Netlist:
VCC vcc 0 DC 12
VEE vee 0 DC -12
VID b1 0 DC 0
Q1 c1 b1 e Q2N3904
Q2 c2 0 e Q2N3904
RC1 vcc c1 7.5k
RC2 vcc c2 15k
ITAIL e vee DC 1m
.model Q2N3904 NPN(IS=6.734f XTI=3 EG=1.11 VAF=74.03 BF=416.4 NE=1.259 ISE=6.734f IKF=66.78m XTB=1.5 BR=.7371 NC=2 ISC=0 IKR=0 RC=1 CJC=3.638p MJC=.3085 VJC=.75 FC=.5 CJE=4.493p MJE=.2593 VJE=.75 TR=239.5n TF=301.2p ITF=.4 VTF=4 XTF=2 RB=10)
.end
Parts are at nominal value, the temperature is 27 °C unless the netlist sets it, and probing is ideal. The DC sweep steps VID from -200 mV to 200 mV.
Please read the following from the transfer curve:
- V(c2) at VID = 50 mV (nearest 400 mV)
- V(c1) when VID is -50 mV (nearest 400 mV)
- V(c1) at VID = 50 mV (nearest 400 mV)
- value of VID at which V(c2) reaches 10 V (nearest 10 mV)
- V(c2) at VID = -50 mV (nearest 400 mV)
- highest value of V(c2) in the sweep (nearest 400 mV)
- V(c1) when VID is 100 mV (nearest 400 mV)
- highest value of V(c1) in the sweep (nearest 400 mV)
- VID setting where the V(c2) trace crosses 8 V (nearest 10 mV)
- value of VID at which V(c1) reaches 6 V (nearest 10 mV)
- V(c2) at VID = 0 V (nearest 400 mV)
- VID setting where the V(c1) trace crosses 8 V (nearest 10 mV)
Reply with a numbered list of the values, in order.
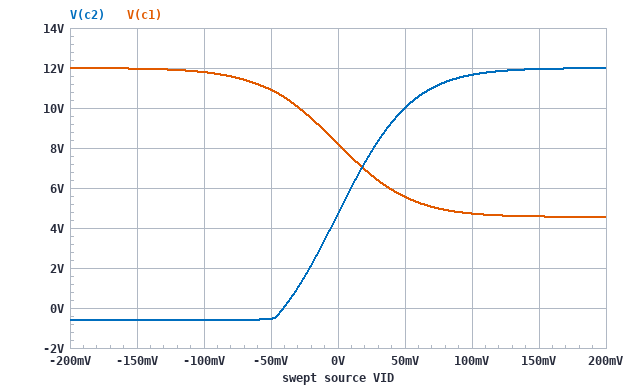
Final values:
1. 10.0 V
2. 10.8 V
3. 5.6 V
4. 50 mV
5. -400 mV
6. 12.0 V
7. 4.8 V
8. 12.0 V
9. 30 mV
10. 40 mV
11. 4.8 V
12. 0 V
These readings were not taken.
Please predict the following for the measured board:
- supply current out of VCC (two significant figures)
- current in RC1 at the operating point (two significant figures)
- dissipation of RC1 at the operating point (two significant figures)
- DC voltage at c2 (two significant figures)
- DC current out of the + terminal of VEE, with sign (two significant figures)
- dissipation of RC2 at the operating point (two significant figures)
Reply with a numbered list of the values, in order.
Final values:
1. 990 µA
2. 510 µA
3. 1.9 mW
4. 4.7 V
5. -1.0 mA
6. 3.5 mW
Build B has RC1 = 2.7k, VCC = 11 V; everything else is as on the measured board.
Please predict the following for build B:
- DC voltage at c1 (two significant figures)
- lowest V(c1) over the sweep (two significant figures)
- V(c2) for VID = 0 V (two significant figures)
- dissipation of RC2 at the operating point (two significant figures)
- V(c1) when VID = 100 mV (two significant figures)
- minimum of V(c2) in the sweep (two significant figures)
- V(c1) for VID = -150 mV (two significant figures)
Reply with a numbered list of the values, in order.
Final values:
1. 9.6 V
2. 8.3 V
3. 3.8 V
4. 3.4 mW
5. 8.4 V
6. -620 mV
7. 11 V
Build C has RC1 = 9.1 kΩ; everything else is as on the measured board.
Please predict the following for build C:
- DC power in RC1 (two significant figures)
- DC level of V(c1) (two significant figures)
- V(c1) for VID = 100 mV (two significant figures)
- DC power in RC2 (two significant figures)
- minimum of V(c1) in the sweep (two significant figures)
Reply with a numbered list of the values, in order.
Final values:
1. 2.3 mW
2. 7.4 V
3. 3.2 V
4. 3.6 mW
5. 3.0 V
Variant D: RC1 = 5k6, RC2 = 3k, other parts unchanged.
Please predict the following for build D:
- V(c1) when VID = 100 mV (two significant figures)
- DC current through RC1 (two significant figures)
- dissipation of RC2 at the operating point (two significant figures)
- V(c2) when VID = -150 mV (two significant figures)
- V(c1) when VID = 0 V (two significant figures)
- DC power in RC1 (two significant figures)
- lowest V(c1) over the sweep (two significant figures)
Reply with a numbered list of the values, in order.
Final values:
1. 6.6 V
2. 490 µA
3. 750 µW
4. 9.0 V
5. 9.2 V
6. 1.4 mW
7. 6.4 V
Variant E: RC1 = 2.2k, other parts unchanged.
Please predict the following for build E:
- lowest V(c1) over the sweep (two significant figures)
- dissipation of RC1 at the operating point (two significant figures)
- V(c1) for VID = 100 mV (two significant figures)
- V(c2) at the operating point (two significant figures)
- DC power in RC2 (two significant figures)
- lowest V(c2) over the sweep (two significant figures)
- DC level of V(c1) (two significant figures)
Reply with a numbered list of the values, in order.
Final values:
1. 9.8 V
2. 580 µW
3. 9.9 V
4. 4.8 V
5. 3.4 mW
6. -610 mV
7. 11 V
